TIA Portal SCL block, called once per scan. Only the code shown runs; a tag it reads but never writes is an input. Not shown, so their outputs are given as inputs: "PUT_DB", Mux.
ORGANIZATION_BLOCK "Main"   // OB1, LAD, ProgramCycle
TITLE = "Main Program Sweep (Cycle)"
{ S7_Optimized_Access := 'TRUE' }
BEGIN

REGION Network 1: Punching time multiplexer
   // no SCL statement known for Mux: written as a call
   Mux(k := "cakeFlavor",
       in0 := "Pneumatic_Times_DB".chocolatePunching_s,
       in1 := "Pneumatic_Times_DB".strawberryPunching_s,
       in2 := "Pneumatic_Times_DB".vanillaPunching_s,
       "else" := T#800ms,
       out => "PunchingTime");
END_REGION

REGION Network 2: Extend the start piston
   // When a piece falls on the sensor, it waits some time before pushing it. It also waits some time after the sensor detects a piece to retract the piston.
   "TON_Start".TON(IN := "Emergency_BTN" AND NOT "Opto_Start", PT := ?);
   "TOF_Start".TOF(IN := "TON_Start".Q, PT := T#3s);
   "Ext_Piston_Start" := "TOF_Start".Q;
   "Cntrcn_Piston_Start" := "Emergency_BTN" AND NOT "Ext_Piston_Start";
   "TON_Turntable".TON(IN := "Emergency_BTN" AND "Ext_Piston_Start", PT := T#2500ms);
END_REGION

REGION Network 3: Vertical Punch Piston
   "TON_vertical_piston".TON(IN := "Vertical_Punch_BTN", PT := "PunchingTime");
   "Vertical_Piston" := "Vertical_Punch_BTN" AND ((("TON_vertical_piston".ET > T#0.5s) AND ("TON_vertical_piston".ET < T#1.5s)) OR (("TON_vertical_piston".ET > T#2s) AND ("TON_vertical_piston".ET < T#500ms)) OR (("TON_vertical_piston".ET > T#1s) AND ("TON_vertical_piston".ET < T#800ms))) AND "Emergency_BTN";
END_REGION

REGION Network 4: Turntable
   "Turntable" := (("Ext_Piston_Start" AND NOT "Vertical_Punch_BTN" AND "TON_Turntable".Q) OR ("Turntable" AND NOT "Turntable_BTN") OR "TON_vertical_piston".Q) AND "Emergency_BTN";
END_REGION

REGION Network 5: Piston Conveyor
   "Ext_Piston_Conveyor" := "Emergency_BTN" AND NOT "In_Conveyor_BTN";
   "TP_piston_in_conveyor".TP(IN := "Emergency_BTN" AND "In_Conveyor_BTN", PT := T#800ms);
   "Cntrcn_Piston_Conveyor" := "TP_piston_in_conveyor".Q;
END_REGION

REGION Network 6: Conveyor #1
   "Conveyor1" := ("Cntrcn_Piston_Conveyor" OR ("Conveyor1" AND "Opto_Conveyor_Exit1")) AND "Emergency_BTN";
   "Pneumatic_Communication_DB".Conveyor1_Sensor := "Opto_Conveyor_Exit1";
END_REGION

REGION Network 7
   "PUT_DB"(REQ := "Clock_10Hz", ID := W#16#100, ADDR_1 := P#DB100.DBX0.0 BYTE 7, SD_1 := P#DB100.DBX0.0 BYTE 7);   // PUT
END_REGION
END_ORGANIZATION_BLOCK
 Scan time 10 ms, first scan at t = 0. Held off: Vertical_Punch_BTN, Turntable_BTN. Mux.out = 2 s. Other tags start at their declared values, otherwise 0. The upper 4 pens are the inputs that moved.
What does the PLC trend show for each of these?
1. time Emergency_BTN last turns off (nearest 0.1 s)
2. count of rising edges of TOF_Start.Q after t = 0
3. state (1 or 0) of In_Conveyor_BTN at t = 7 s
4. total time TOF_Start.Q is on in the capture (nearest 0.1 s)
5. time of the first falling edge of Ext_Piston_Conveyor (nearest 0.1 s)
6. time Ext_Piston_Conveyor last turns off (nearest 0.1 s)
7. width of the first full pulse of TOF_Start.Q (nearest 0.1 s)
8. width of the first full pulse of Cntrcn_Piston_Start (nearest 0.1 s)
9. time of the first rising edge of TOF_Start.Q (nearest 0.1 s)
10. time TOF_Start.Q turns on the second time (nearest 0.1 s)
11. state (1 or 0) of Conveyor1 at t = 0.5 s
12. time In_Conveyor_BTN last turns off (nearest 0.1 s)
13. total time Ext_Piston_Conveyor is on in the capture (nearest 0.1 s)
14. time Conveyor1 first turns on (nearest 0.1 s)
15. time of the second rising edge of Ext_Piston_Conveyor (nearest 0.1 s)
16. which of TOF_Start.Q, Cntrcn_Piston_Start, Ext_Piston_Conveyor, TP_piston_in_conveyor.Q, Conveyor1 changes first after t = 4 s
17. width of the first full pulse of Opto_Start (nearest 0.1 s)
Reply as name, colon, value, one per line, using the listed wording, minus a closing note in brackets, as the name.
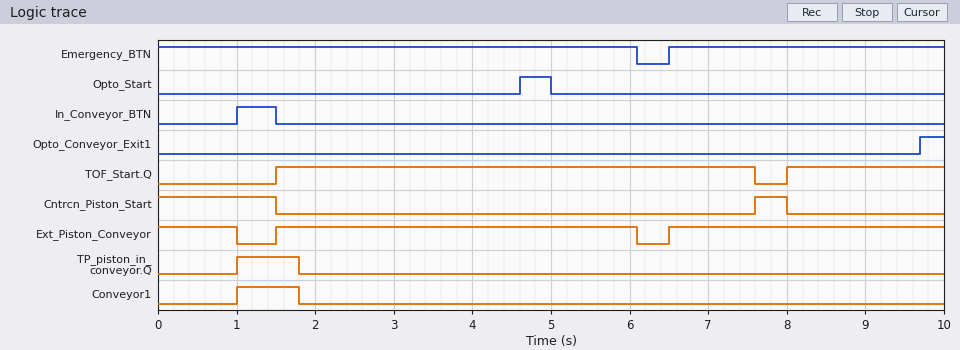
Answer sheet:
time Emergency_BTN last turns off: 6.1 s
count of rising edges of TOF_Start.Q after t = 0: 2
state (1 or 0) of In_Conveyor_BTN at t = 7 s: 0
total time TOF_Start.Q is on in the capture: 8.1 s
time of the first falling edge of Ext_Piston_Conveyor: 1.0 s
time Ext_Piston_Conveyor last turns off: 6.1 s
width of the first full pulse of TOF_Start.Q: 6.1 s
width of the first full pulse of Cntrcn_Piston_Start: 0.4 s
time of the first rising edge of TOF_Start.Q: 1.5 s
time TOF_Start.Q turns on the second time: 8.0 s
state (1 or 0) of Conveyor1 at t = 0.5 s: 0
time In_Conveyor_BTN last turns off: 1.5 s
total time Ext_Piston_Conveyor is on in the capture: 9.1 s
time Conveyor1 first turns on: 1.0 s
time of the second rising edge of Ext_Piston_Conveyor: 6.5 s
which of TOF_Start.Q, Cntrcn_Piston_Start, Ext_Piston_Conveyor, TP_piston_in_conveyor.Q, Conveyor1 changes first after t = 4 s: Ext_Piston_Conveyor
width of the first full pulse of Opto_Start: 0.4 s
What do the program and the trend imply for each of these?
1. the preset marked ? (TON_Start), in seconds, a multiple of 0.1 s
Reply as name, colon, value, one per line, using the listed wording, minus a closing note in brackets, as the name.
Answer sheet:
the preset marked ? (TON_Start), in seconds, a multiple of 0.1 s: 1.5 s
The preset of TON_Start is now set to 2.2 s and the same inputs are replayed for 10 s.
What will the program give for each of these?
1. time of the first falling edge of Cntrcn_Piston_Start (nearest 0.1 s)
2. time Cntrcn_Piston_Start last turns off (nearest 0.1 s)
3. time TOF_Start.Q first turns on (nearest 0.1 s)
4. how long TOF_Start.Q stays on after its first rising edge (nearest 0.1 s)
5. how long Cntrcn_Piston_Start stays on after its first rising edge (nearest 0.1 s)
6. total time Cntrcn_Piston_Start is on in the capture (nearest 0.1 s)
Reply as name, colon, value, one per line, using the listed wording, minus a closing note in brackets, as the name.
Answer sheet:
time of the first falling edge of Cntrcn_Piston_Start: 2.2 s
time Cntrcn_Piston_Start last turns off: 8.7 s
time TOF_Start.Q first turns on: 2.2 s
how long TOF_Start.Q stays on after its first rising edge: 5.4 s
how long Cntrcn_Piston_Start stays on after its first rising edge: 1.1 s
total time Cntrcn_Piston_Start is on in the capture: 3.3 s
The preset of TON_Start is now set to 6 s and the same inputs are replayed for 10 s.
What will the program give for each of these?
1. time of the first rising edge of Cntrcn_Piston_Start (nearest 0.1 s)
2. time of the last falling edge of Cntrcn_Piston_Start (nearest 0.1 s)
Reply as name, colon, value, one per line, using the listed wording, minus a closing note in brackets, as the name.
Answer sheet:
time of the first rising edge of Cntrcn_Piston_Start: 6.5 s
time of the last falling edge of Cntrcn_Piston_Start: 6.1 s
